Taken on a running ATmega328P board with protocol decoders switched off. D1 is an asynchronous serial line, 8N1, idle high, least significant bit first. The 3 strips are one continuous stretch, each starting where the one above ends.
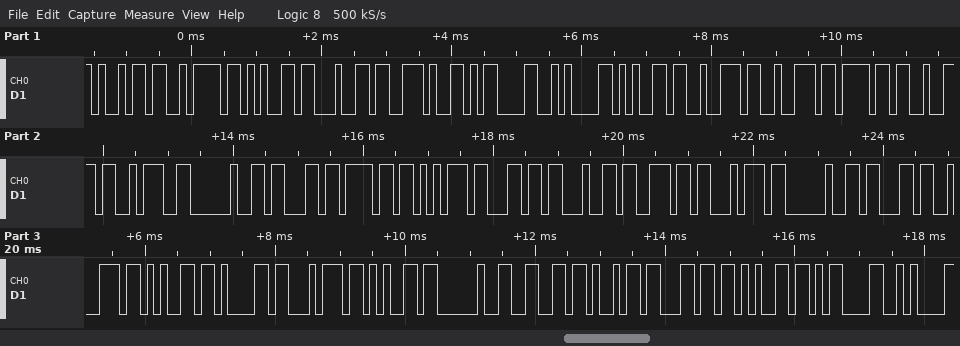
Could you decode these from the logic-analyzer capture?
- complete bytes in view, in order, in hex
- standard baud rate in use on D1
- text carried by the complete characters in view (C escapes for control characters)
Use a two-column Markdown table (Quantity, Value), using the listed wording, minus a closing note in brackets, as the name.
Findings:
| Quantity | Value |
|---|---|
| complete bytes in view, in order, in hex | 69 7A 65 64 2E 0D 0A 65 72 72 6F 72 3A 20 63 6F 75 6C 64 6E 74 20 63 72 65 61 74 65 20 66 69 6C 65 0D 0A |
| standard baud rate in use on D1 | 9600 baud |
| text carried by the complete characters in view | "ized.\r\nerror: couldnt create file\r\n" |
